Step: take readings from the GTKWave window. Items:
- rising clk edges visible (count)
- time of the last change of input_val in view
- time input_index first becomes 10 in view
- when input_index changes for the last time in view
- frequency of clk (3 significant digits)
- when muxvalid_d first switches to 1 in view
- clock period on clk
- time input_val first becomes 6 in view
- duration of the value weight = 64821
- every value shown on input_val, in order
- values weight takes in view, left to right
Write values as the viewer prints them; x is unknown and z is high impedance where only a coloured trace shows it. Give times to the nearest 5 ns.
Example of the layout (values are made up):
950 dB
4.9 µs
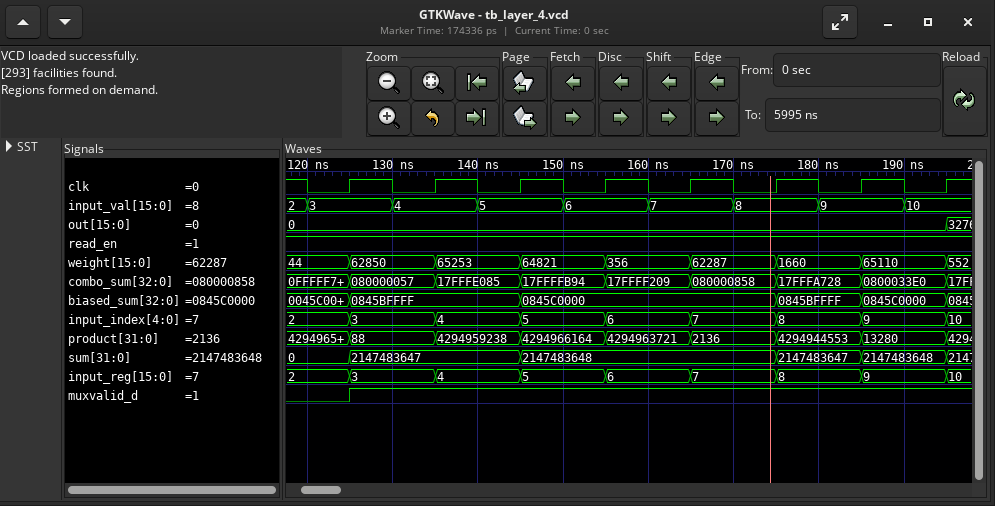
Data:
8
190 ns
195 ns
195 ns
100 MHz
125 ns
10 ns
150 ns
10 ns
2, 3, 4, 5, 6, 7, 8, 9, 10
44, 62850, 65253, 64821, 356, 62287, 1660, 65110, 552
